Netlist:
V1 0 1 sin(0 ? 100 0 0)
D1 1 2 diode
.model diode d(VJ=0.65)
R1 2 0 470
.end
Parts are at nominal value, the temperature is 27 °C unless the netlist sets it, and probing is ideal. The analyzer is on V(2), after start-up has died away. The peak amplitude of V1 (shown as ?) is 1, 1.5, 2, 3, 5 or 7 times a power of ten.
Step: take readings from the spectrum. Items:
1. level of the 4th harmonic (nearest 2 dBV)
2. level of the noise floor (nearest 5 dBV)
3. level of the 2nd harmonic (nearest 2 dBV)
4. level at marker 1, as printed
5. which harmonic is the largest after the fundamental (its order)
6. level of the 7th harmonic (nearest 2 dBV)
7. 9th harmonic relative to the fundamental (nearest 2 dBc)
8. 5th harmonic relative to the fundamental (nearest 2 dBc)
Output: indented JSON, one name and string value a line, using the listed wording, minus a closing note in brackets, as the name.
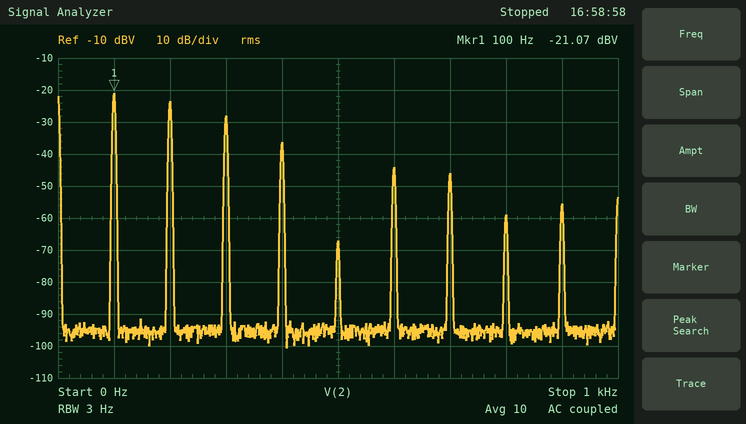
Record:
{
  "level of the 4th harmonic": "-36 dBV",
  "level of the noise floor": "-95 dBV",
  "level of the 2nd harmonic": "-24 dBV",
  "level at marker 1, as printed": "-21.07 dBV",
  "which harmonic is the largest after the fundamental": "2",
  "level of the 7th harmonic": "-46 dBV",
  "9th harmonic relative to the fundamental": "-34 dBc",
  "5th harmonic relative to the fundamental": "-46 dBc"
}
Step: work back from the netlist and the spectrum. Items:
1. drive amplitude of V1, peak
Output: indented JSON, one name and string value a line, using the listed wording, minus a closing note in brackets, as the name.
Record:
{
  "drive amplitude of V1, peak": "1 V"
}
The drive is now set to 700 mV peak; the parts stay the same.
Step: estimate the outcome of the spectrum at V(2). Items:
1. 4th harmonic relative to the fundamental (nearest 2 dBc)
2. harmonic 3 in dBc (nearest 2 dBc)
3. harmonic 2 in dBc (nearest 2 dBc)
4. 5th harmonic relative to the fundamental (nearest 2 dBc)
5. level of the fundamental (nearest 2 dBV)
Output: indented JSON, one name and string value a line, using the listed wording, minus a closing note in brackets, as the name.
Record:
{
  "4th harmonic relative to the fundamental": "-6 dBc",
  "harmonic 3 in dBc": "-4 dBc",
  "harmonic 2 in dBc": "-2 dBc",
  "5th harmonic relative to the fundamental": "-10 dBc",
  "level of the fundamental": "-36 dBV"
}
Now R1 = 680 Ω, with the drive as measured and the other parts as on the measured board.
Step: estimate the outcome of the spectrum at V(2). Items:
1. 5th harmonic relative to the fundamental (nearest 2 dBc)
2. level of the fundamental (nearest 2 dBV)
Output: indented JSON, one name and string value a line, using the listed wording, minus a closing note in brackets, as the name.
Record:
{
  "5th harmonic relative to the fundamental": "-38 dBc",
  "level of the fundamental": "-20 dBV"
}
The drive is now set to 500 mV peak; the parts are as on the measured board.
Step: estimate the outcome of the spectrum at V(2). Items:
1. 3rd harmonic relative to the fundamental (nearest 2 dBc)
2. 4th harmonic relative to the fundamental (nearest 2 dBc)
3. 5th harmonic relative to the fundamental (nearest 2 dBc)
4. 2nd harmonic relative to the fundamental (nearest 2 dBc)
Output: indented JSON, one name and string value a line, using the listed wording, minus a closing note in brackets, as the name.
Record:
{
  "3rd harmonic relative to the fundamental": "-2 dBc",
  "4th harmonic relative to the fundamental": "-4 dBc",
  "5th harmonic relative to the fundamental": "-6 dBc",
  "2nd harmonic relative to the fundamental": "0 dBc"
}
